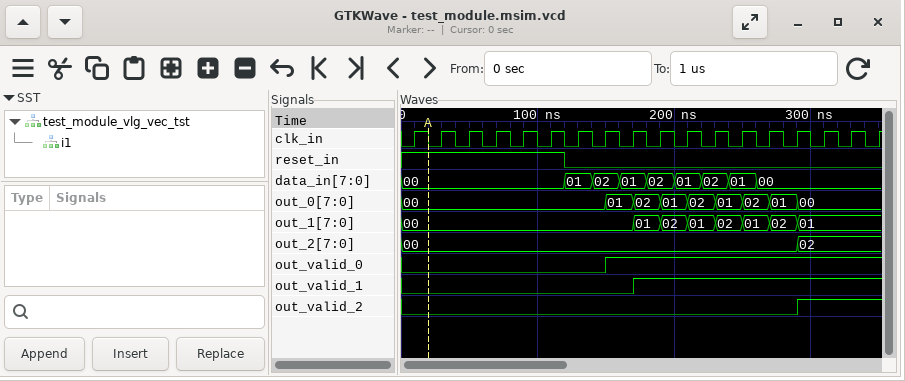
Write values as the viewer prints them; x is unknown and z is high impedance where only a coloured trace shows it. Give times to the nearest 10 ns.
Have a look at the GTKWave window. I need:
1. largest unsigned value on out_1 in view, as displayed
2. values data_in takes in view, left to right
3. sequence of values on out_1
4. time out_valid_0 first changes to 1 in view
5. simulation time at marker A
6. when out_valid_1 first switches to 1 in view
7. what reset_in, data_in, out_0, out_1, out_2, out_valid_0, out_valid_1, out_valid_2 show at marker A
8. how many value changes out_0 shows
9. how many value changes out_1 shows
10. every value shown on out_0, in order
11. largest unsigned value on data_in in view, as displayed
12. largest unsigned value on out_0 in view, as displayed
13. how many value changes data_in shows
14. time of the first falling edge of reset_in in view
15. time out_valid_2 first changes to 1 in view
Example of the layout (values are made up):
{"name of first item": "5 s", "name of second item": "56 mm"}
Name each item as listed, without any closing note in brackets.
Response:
{"largest unsigned value on out_1 in view, as displayed": "02", "values data_in takes in view, left to right": "00, 01, 02, 01, 02, 01, 02, 01, 00", "sequence of values on out_1": "00, 01, 02, 01, 02, 01, 02, 01", "time out_valid_0 first changes to 1 in view": "150 ns", "simulation time at marker A": "20 ns", "when out_valid_1 first switches to 1 in view": "170 ns", "what reset_in, data_in, out_0, out_1, out_2, out_valid_0, out_valid_1, out_valid_2 show at marker A": "reset_in=1, data_in=00, out_0=00, out_1=00, out_2=00, out_valid_0=0, out_valid_1=0, out_valid_2=0", "how many value changes out_0 shows": "8", "how many value changes out_1 shows": "7", "every value shown on out_0, in order": "00, 01, 02, 01, 02, 01, 02, 01, 00", "largest unsigned value on data_in in view, as displayed": "02", "largest unsigned value on out_0 in view, as displayed": "02", "how many value changes data_in shows": "8", "time of the first falling edge of reset_in in view": "120 ns", "time out_valid_2 first changes to 1 in view": "290 ns"}
